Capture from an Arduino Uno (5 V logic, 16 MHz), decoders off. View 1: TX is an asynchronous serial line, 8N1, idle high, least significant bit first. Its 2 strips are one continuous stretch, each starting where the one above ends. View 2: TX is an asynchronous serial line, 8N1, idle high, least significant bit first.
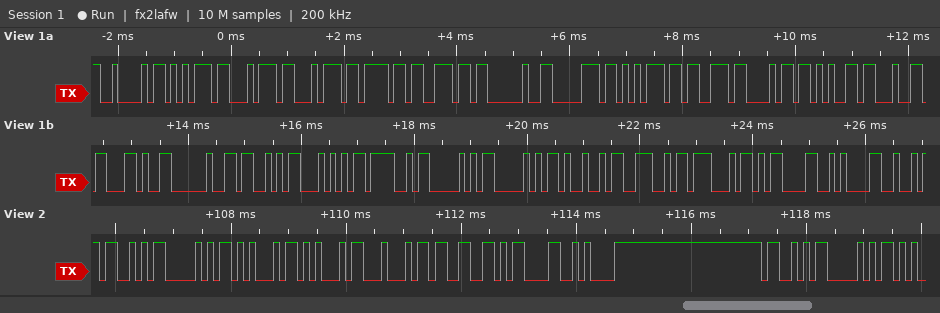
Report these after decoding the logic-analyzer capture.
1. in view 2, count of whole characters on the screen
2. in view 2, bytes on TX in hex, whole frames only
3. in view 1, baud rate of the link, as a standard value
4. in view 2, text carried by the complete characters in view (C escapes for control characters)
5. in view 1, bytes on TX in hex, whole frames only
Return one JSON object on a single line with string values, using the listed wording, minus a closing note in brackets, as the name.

{"in view 2, count of whole characters on the screen": "10", "in view 2, bytes on TX in hex, whole frames only": "53 50 45 45 44 33 0D 0A 53 50", "in view 1, baud rate of the link, as a standard value": "9600 baud", "in view 2, text carried by the complete characters in view": "\"SPEED3\\r\\nSP\"", "in view 1, bytes on TX in hex, whole frames only": "42 75 74 74 6F 6E 20 70 75 73 68 65 64 2C 20 53 54 4F 50 50 49 4E 47 0D 0A"}
